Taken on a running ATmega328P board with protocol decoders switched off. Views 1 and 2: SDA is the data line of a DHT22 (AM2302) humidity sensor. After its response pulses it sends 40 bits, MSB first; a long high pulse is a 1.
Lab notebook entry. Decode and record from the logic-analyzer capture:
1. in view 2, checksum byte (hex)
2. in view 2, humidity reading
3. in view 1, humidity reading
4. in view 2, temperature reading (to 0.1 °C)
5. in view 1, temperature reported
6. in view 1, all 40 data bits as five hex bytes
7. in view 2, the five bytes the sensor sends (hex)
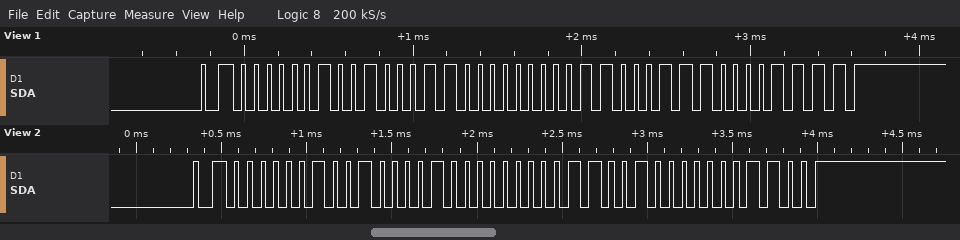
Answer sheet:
0x0C
57.8 %
58.2 %
20.0 °C
19.9 °C
02 46 00 C7 0F
02 42 00 C8 0C
